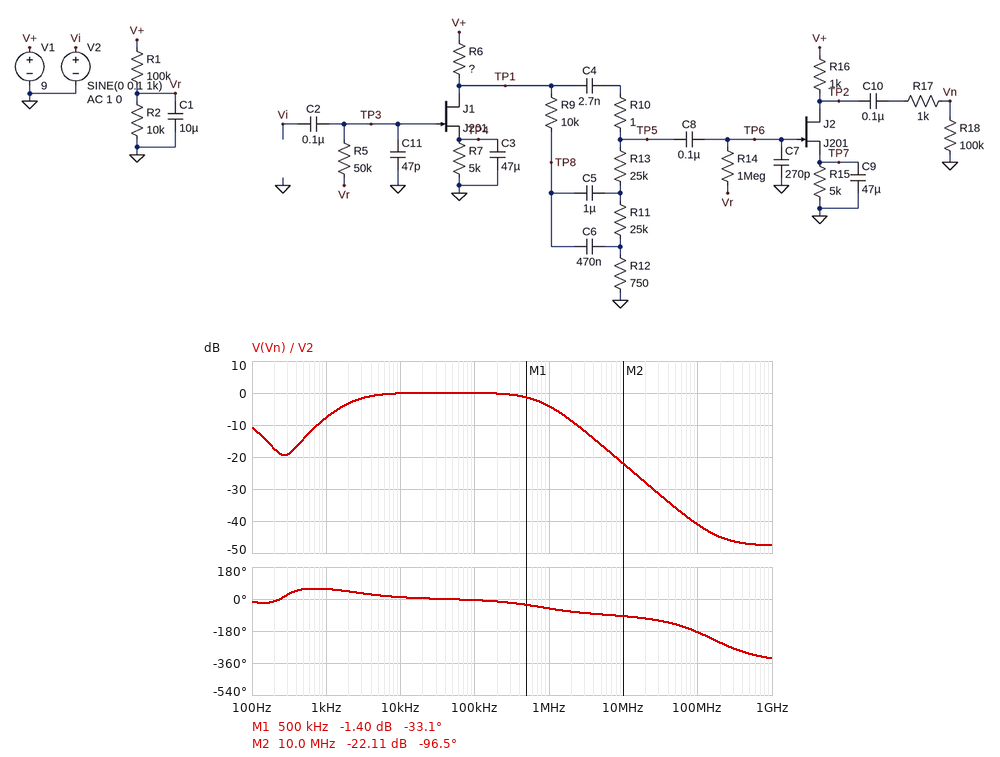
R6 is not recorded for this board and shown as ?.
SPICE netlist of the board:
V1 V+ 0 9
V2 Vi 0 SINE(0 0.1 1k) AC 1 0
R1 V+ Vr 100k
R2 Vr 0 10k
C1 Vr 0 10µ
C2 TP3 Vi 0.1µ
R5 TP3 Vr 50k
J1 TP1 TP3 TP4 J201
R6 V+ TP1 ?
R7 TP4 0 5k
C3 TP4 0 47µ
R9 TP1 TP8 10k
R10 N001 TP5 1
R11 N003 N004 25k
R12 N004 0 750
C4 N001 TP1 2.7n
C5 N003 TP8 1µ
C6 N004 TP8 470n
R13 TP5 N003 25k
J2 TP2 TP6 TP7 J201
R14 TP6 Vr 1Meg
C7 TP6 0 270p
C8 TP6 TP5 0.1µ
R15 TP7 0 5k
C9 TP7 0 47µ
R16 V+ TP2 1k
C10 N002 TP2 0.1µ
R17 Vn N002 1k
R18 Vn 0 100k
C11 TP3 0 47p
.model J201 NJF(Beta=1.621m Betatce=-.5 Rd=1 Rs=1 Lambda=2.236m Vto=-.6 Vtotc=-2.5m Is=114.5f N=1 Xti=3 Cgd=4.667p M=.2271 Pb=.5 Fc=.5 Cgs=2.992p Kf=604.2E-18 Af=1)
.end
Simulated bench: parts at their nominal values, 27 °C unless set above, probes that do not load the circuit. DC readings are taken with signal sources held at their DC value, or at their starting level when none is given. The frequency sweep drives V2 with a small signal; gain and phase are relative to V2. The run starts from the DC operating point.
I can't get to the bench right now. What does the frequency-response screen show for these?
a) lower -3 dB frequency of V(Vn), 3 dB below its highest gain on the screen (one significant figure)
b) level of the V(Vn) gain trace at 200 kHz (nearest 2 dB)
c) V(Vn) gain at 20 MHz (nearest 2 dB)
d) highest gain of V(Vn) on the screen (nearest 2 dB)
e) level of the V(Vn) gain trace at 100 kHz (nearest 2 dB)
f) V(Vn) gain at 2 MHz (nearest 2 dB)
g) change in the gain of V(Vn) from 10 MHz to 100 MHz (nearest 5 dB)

2 kHz
0 dB
-28 dB
0 dB
0 dB
-8 dB
-20 dB
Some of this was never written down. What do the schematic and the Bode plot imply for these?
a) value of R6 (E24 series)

910 Ω
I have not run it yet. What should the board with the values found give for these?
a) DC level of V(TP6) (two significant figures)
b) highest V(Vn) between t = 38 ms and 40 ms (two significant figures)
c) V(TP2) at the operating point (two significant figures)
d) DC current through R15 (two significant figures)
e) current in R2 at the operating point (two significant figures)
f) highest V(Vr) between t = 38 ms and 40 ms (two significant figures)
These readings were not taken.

820 mV
42 mV
8.8 V
210 µA
82 µA
820 mV
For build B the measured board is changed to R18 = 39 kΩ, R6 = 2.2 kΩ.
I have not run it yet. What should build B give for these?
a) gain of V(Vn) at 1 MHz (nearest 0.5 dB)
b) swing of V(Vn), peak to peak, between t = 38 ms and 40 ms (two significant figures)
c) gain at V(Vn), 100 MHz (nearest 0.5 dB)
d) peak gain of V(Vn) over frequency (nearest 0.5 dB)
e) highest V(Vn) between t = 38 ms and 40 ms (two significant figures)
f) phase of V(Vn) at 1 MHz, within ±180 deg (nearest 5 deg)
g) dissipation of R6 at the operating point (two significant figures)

-3.0 dB
170 mV
-41.5 dB
6.5 dB
85 mV
-70 deg
99 µW
